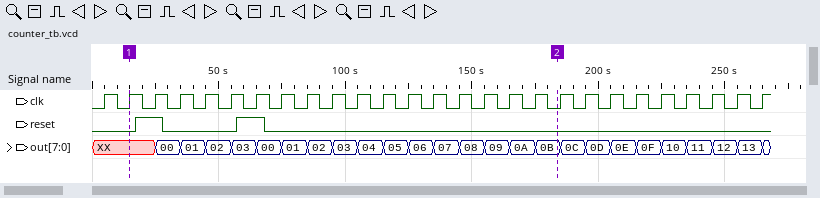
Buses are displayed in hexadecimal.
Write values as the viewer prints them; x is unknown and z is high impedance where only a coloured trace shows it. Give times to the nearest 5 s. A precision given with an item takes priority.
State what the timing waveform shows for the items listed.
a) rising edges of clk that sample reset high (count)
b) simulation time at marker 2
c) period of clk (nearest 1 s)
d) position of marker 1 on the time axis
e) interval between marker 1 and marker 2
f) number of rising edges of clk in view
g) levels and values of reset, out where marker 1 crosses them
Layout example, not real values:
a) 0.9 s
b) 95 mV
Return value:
a) 2
b) 185 s
c) 10 s
d) 15 s
e) 170 s
f) 27
g) reset=0, out=XX
